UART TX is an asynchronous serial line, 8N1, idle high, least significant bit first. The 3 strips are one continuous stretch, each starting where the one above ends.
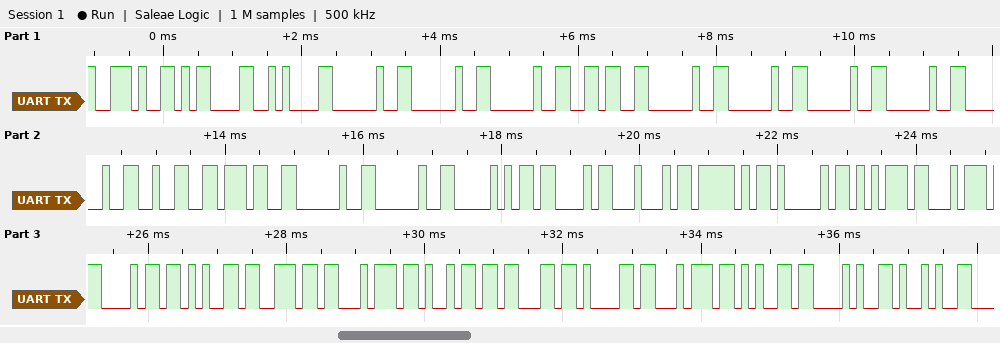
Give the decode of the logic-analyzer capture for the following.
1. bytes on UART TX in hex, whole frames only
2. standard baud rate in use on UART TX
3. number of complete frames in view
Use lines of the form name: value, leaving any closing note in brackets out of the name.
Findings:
bytes on UART TX in hex, whole frames only: 2E 0D 0A 20 20 20 36 20 20 20 20 20 32 37 20 20 50 43 44 5F 41 75 74 68 65 6E 74 69 63 61 74 65 28 29
standard baud rate in use on UART TX: 9600 baud
number of complete frames in view: 34
